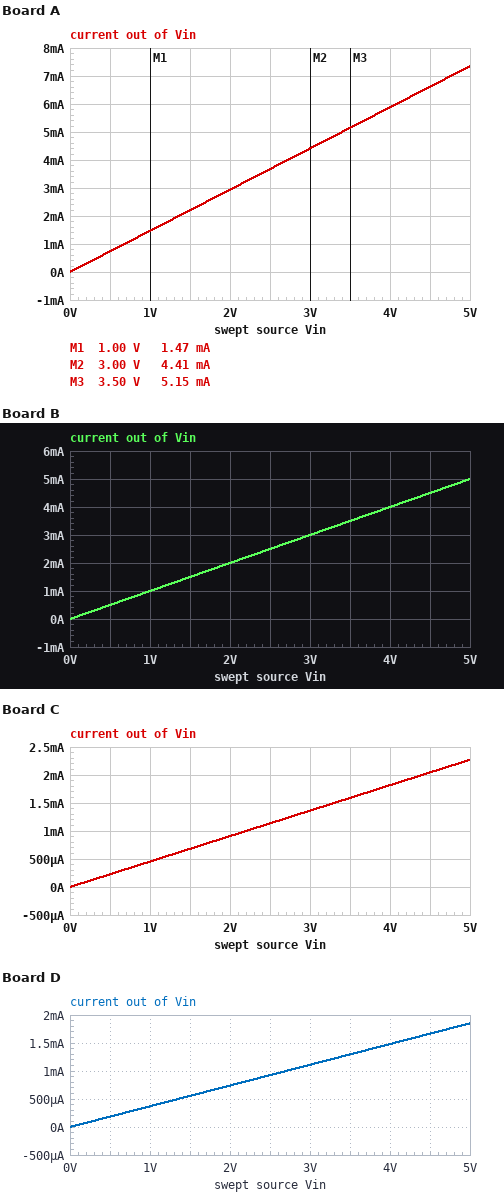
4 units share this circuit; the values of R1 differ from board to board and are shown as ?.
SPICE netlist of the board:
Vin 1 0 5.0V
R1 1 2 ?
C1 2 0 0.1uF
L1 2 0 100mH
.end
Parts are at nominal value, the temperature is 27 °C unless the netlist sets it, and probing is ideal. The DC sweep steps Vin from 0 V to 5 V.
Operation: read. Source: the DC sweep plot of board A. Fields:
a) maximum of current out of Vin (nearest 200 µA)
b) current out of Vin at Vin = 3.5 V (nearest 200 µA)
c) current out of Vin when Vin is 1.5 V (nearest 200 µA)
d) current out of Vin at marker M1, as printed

7.4 mA
5.2 mA
2.2 mA
1.47 mA
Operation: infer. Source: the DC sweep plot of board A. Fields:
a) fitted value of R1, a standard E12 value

680 Ω
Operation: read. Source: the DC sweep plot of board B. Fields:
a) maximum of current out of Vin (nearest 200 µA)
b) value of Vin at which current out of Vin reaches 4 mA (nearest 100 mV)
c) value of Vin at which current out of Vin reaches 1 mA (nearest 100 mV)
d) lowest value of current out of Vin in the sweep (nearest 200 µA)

5.0 mA
4.0 V
1.0 V
0 A
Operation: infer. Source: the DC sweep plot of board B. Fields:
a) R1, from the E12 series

1 kΩ
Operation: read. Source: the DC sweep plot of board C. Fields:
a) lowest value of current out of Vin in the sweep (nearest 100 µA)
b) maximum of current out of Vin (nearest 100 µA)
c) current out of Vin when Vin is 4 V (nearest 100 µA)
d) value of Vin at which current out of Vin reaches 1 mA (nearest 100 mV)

0 A
2.3 mA
1.8 mA
2.2 V
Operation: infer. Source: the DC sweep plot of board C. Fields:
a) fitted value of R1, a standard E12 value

2.2 kΩ
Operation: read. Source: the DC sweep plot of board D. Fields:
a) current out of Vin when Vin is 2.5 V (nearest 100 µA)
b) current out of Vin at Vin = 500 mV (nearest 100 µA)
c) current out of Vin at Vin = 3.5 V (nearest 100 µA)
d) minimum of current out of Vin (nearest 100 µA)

900 µA
200 µA
1.3 mA
0 A
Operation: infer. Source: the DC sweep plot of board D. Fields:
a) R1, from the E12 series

2.7 kΩ
